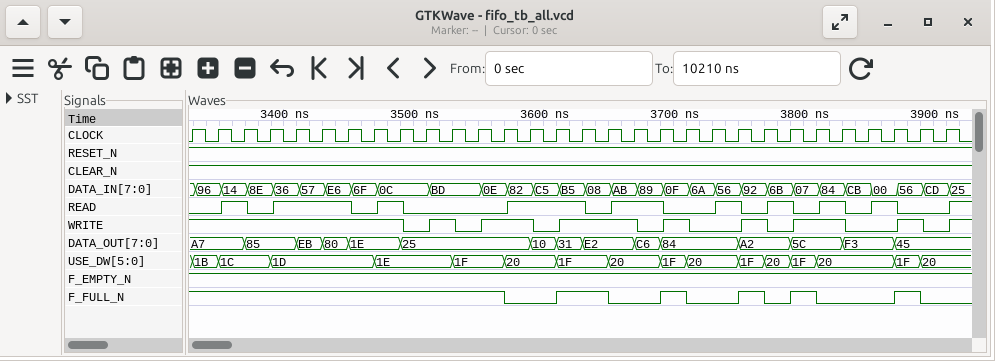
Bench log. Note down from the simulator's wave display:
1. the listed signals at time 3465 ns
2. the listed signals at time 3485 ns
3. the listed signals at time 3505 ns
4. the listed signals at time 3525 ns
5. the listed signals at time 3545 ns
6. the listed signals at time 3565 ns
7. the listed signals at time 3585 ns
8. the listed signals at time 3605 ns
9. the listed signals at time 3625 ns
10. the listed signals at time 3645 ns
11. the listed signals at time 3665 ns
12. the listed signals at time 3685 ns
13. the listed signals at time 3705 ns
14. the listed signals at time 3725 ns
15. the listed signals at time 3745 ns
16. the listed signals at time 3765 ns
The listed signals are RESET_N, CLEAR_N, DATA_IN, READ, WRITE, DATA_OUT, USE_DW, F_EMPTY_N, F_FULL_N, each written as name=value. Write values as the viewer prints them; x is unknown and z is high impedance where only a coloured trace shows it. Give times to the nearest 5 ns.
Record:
RESET_N=1, CLEAR_N=1, DATA_IN=6F, READ=0, WRITE=1, DATA_OUT=1E, USE_DW=1D, F_EMPTY_N=1, F_FULL_N=1
RESET_N=1, CLEAR_N=1, DATA_IN=0C, READ=1, WRITE=1, DATA_OUT=1E, USE_DW=1E, F_EMPTY_N=1, F_FULL_N=1
RESET_N=1, CLEAR_N=1, DATA_IN=0C, READ=0, WRITE=0, DATA_OUT=25, USE_DW=1E, F_EMPTY_N=1, F_FULL_N=1
RESET_N=1, CLEAR_N=1, DATA_IN=BD, READ=0, WRITE=1, DATA_OUT=25, USE_DW=1E, F_EMPTY_N=1, F_FULL_N=1
RESET_N=1, CLEAR_N=1, DATA_IN=BD, READ=0, WRITE=0, DATA_OUT=25, USE_DW=1F, F_EMPTY_N=1, F_FULL_N=1
RESET_N=1, CLEAR_N=1, DATA_IN=0E, READ=0, WRITE=1, DATA_OUT=25, USE_DW=1F, F_EMPTY_N=1, F_FULL_N=1
RESET_N=1, CLEAR_N=1, DATA_IN=82, READ=1, WRITE=1, DATA_OUT=25, USE_DW=20, F_EMPTY_N=1, F_FULL_N=0
RESET_N=1, CLEAR_N=1, DATA_IN=C5, READ=1, WRITE=0, DATA_OUT=10, USE_DW=20, F_EMPTY_N=1, F_FULL_N=0
RESET_N=1, CLEAR_N=1, DATA_IN=B5, READ=1, WRITE=1, DATA_OUT=31, USE_DW=1F, F_EMPTY_N=1, F_FULL_N=1
RESET_N=1, CLEAR_N=1, DATA_IN=08, READ=0, WRITE=1, DATA_OUT=E2, USE_DW=1F, F_EMPTY_N=1, F_FULL_N=1
RESET_N=1, CLEAR_N=1, DATA_IN=AB, READ=1, WRITE=1, DATA_OUT=E2, USE_DW=20, F_EMPTY_N=1, F_FULL_N=0
RESET_N=1, CLEAR_N=1, DATA_IN=89, READ=1, WRITE=0, DATA_OUT=C6, USE_DW=20, F_EMPTY_N=1, F_FULL_N=0
RESET_N=1, CLEAR_N=1, DATA_IN=0F, READ=0, WRITE=1, DATA_OUT=84, USE_DW=1F, F_EMPTY_N=1, F_FULL_N=1
RESET_N=1, CLEAR_N=1, DATA_IN=6A, READ=0, WRITE=0, DATA_OUT=84, USE_DW=20, F_EMPTY_N=1, F_FULL_N=0
RESET_N=1, CLEAR_N=1, DATA_IN=56, READ=1, WRITE=0, DATA_OUT=84, USE_DW=20, F_EMPTY_N=1, F_FULL_N=0
RESET_N=1, CLEAR_N=1, DATA_IN=92, READ=0, WRITE=1, DATA_OUT=A2, USE_DW=1F, F_EMPTY_N=1, F_FULL_N=1
